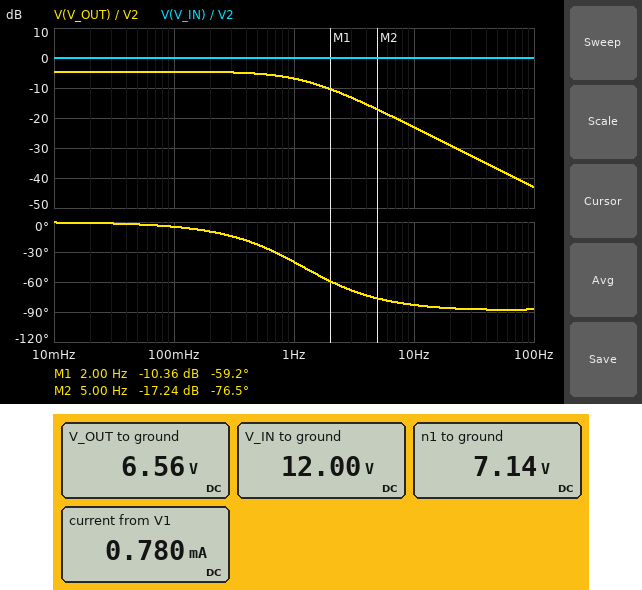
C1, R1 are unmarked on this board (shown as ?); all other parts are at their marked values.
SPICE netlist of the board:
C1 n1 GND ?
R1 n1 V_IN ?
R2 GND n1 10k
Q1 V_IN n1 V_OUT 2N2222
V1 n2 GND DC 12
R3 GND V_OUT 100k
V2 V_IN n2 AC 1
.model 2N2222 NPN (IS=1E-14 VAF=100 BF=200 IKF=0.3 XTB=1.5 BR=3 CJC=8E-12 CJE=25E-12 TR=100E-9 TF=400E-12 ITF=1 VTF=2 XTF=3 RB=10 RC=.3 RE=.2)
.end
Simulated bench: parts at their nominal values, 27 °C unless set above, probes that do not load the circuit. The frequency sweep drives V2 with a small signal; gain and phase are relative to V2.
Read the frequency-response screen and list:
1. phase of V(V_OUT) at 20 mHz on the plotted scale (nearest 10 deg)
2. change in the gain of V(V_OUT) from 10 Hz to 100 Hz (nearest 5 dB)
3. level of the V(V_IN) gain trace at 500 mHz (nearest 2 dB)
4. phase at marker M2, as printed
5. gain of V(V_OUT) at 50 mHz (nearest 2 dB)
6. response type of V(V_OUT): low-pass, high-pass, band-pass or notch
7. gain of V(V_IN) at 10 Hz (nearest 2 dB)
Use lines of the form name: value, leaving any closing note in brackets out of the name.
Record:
phase of V(V_OUT) at 20 mHz on the plotted scale: 0 deg
change in the gain of V(V_OUT) from 10 Hz to 100 Hz: -20 dB
level of the V(V_IN) gain trace at 500 mHz: 0 dB
phase at marker M2, as printed: -76.5 deg
gain of V(V_OUT) at 50 mHz: -4 dB
response type of V(V_OUT): low-pass, high-pass, band-pass or notch: low-pass
gain of V(V_IN) at 10 Hz: 0 dB
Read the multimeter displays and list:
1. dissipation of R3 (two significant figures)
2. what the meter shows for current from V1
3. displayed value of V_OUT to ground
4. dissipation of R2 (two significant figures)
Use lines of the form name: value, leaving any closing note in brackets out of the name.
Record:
dissipation of R3: 430 µW
what the meter shows for current from V1: 0.780 mA
displayed value of V_OUT to ground: 6.56 V
dissipation of R2: 5.1 mW
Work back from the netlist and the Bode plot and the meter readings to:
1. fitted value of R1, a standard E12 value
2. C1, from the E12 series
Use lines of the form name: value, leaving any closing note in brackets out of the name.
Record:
fitted value of R1, a standard E12 value: 6.8 kΩ
C1, from the E12 series: 33 µF
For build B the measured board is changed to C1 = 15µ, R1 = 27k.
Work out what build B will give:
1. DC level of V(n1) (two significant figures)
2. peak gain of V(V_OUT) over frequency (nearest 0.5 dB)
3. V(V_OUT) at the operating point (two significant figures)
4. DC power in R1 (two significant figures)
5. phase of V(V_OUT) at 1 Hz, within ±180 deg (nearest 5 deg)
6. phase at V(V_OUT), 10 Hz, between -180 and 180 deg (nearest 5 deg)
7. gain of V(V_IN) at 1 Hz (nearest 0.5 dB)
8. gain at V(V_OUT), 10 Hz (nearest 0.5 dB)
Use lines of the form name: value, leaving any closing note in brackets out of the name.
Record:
DC level of V(n1): 3.2 V
peak gain of V(V_OUT) over frequency: -11.5 dB
V(V_OUT) at the operating point: 2.7 V
DC power in R1: 2.8 mW
phase of V(V_OUT) at 1 Hz, within ±180 deg: -35 deg
phase at V(V_OUT), 10 Hz, between -180 and 180 deg: -80 deg
gain of V(V_IN) at 1 Hz: 0 dB
gain at V(V_OUT), 10 Hz: -28.5 dB
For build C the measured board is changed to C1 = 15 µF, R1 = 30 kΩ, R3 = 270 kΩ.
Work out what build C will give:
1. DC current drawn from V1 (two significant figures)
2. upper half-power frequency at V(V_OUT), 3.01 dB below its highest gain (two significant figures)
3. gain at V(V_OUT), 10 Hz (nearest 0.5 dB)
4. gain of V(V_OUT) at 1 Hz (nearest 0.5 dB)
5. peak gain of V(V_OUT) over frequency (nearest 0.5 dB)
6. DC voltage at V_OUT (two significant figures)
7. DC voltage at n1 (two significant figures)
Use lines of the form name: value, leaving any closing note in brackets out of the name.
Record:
DC current drawn from V1: 310 µA
upper half-power frequency at V(V_OUT), 3.01 dB below its highest gain: 1.4 Hz
gain at V(V_OUT), 10 Hz: -29.0 dB
gain of V(V_OUT) at 1 Hz: -14.0 dB
peak gain of V(V_OUT) over frequency: -12.0 dB
DC voltage at V_OUT: 2.5 V
DC voltage at n1: 3.0 V
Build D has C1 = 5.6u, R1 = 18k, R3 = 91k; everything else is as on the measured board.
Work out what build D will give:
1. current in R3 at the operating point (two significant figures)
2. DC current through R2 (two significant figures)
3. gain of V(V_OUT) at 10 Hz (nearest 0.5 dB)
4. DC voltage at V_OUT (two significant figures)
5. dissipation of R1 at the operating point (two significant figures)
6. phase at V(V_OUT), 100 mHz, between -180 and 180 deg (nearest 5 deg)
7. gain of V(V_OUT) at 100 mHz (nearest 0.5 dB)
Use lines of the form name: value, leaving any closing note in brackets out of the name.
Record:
current in R3 at the operating point: 41 µA
DC current through R2: 430 µA
gain of V(V_OUT) at 10 Hz: -17.0 dB
DC voltage at V_OUT: 3.7 V
dissipation of R1 at the operating point: 3.3 mW
phase at V(V_OUT), 100 mHz, between -180 and 180 deg: 0 deg
gain of V(V_OUT) at 100 mHz: -9.0 dB
